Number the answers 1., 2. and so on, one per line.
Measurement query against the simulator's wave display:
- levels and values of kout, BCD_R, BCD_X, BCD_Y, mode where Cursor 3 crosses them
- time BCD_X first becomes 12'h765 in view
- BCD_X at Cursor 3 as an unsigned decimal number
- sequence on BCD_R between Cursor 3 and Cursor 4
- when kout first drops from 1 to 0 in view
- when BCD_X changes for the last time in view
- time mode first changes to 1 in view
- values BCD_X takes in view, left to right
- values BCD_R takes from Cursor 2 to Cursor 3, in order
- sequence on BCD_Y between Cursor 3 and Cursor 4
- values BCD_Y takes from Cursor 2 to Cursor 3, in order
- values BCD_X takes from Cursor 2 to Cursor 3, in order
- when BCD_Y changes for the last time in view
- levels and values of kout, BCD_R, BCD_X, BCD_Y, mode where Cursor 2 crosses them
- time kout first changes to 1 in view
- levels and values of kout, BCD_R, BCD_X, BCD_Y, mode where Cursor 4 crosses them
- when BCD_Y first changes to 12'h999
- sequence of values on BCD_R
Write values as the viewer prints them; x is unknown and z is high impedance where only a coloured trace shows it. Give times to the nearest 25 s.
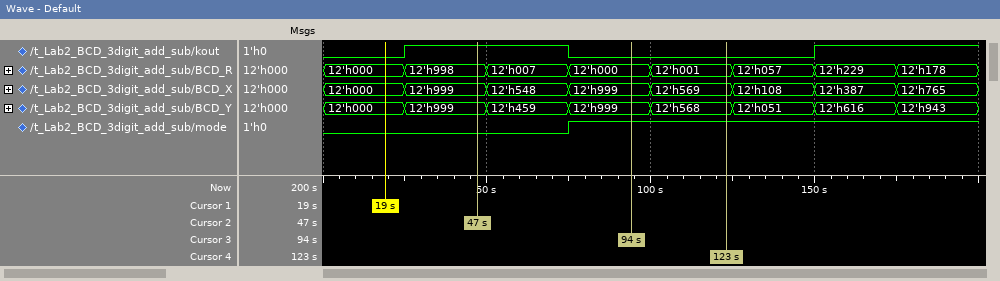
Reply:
1. kout=0, BCD_R=12'h000, BCD_X=12'h999, BCD_Y=12'h999, mode=1
2. 175 s
3. 2457
4. 12'h000, 12'h001
5. 75 s
6. 175 s
7. 75 s
8. 12'h000, 12'h999, 12'h548, 12'h999, 12'h569, 12'h108, 12'h387, 12'h765
9. 12'h998, 12'h007, 12'h000
10. 12'h999, 12'h568
11. 12'h999, 12'h459, 12'h999
12. 12'h999, 12'h548, 12'h999
13. 175 s
14. kout=1, BCD_R=12'h998, BCD_X=12'h999, BCD_Y=12'h999, mode=0
15. 25 s
16. kout=0, BCD_R=12'h001, BCD_X=12'h569, BCD_Y=12'h568, mode=1
17. 25 s
18. 12'h000, 12'h998, 12'h007, 12'h000, 12'h001, 12'h057, 12'h229, 12'h178
